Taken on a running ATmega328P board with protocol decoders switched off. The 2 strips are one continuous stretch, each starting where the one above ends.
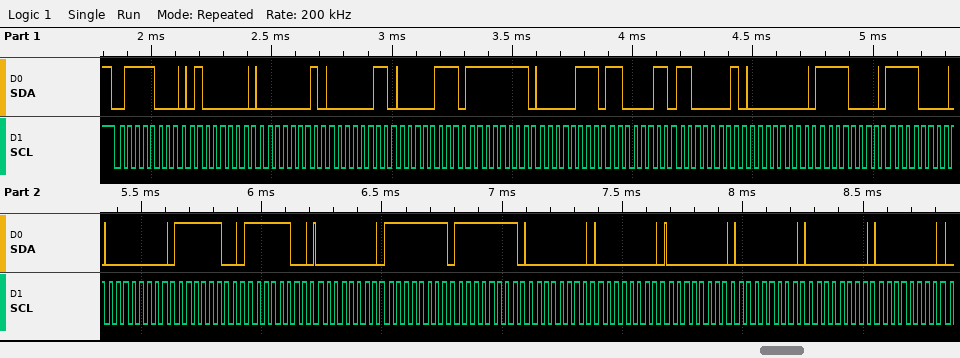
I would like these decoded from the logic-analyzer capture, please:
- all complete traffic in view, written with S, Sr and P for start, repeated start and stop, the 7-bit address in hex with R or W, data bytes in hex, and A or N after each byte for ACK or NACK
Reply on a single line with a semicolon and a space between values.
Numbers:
S 3CW A 40 A 01 A 03 A 07 A FF A 07 A C3 A C1 A 00 A F0 A F0 A 00 A FC A FC A 00 A FF A FF A 00 A 00 A 00 A 00 A 00 A 00 A
